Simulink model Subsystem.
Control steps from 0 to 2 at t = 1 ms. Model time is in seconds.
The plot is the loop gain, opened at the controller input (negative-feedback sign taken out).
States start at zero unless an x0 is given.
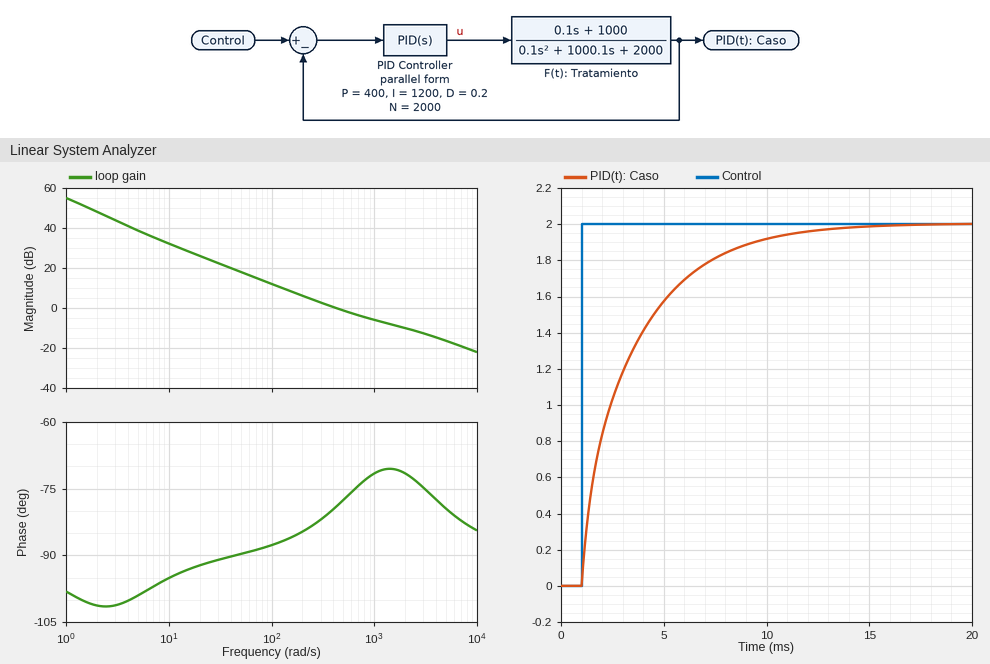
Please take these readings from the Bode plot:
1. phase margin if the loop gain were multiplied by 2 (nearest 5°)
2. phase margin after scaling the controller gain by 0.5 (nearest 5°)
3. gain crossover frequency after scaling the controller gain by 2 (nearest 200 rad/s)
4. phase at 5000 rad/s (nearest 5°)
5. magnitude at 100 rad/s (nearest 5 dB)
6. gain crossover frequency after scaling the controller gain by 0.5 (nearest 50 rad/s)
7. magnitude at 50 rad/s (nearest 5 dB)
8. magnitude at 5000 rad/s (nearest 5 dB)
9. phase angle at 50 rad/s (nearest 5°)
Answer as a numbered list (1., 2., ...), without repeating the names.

1. 110°
2. 95°
3. 1000 rad/s
4. -80°
5. 10 dB
6. 200 rad/s
7. 20 dB
8. -15 dB
9. -90°
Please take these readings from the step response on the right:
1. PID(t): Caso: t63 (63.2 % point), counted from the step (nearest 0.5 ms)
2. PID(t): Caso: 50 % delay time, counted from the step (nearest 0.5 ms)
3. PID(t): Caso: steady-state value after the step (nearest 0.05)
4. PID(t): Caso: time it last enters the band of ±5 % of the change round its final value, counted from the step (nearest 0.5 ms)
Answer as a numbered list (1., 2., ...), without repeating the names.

1. 2.5 ms
2. 1.5 ms
3. 2.00
4. 8.5 ms
